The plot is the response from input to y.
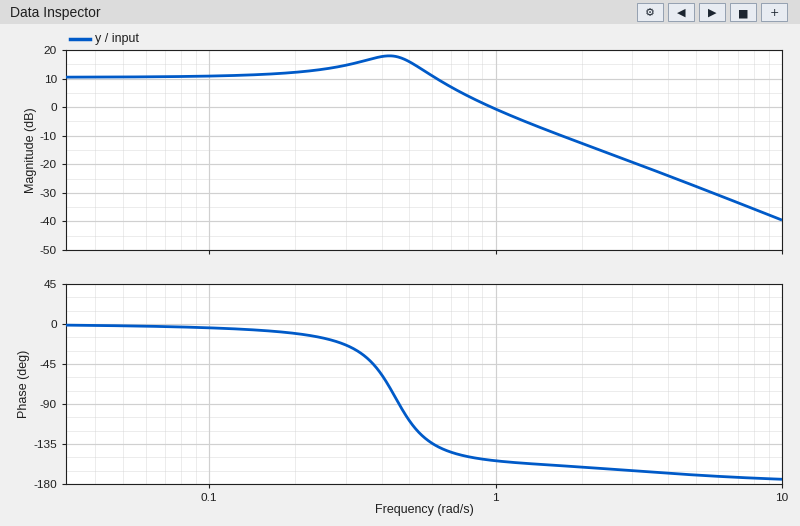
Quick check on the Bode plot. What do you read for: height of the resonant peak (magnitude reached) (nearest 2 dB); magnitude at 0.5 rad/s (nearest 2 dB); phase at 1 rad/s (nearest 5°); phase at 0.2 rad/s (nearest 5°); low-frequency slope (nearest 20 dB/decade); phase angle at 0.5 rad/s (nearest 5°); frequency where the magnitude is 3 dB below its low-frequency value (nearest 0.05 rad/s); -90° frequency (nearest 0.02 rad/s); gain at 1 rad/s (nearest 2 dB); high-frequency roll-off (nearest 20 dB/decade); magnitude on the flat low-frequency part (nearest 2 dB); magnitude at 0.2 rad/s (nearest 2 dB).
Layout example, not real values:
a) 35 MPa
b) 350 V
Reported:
a) 18 dB
b) 16 dB
c) -155°
d) -10°
e) 0 dB/decade
f) -110°
g) 0.70 rad/s
h) 0.46 rad/s
i) 0 dB
j) -40 dB/decade
k) 10 dB
l) 12 dB
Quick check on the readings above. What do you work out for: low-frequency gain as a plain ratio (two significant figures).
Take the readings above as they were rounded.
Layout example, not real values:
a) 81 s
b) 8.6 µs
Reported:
a) 3.2
